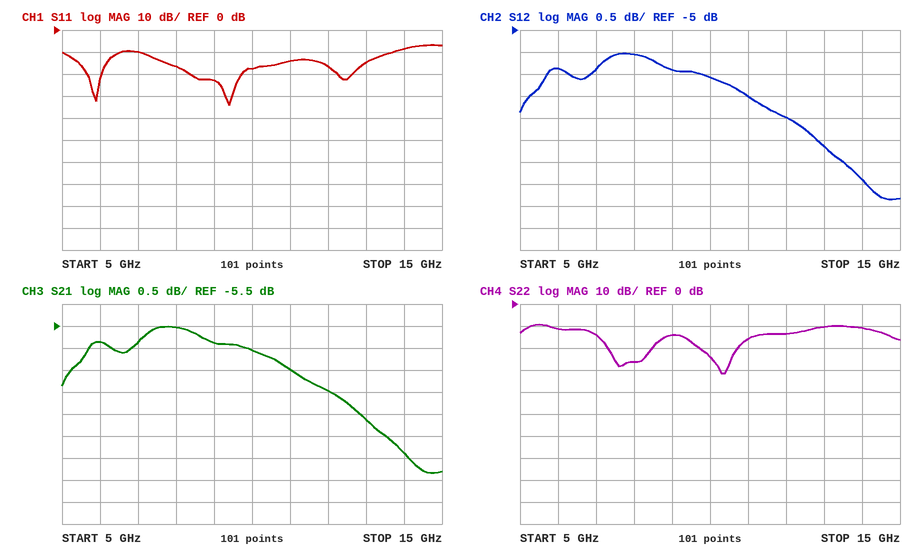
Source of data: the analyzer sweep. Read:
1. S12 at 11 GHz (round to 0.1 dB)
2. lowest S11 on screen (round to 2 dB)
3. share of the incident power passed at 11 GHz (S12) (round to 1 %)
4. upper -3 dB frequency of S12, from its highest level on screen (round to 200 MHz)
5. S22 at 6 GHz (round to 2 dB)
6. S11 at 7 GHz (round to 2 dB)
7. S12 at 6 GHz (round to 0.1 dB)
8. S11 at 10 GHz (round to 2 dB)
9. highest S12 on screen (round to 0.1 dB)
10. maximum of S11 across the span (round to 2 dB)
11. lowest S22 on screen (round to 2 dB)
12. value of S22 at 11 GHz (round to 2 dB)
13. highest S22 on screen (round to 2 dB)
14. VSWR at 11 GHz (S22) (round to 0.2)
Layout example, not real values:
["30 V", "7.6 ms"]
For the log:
["-6.5 dB", "-34 dB", "22 %", "14.2 GHz", "-12 dB", "-10 dB", "-5.9 dB", "-18 dB", "-5.5 dB", "-6 dB", "-32 dB", "-16 dB", "-10 dB", "1.4"]
